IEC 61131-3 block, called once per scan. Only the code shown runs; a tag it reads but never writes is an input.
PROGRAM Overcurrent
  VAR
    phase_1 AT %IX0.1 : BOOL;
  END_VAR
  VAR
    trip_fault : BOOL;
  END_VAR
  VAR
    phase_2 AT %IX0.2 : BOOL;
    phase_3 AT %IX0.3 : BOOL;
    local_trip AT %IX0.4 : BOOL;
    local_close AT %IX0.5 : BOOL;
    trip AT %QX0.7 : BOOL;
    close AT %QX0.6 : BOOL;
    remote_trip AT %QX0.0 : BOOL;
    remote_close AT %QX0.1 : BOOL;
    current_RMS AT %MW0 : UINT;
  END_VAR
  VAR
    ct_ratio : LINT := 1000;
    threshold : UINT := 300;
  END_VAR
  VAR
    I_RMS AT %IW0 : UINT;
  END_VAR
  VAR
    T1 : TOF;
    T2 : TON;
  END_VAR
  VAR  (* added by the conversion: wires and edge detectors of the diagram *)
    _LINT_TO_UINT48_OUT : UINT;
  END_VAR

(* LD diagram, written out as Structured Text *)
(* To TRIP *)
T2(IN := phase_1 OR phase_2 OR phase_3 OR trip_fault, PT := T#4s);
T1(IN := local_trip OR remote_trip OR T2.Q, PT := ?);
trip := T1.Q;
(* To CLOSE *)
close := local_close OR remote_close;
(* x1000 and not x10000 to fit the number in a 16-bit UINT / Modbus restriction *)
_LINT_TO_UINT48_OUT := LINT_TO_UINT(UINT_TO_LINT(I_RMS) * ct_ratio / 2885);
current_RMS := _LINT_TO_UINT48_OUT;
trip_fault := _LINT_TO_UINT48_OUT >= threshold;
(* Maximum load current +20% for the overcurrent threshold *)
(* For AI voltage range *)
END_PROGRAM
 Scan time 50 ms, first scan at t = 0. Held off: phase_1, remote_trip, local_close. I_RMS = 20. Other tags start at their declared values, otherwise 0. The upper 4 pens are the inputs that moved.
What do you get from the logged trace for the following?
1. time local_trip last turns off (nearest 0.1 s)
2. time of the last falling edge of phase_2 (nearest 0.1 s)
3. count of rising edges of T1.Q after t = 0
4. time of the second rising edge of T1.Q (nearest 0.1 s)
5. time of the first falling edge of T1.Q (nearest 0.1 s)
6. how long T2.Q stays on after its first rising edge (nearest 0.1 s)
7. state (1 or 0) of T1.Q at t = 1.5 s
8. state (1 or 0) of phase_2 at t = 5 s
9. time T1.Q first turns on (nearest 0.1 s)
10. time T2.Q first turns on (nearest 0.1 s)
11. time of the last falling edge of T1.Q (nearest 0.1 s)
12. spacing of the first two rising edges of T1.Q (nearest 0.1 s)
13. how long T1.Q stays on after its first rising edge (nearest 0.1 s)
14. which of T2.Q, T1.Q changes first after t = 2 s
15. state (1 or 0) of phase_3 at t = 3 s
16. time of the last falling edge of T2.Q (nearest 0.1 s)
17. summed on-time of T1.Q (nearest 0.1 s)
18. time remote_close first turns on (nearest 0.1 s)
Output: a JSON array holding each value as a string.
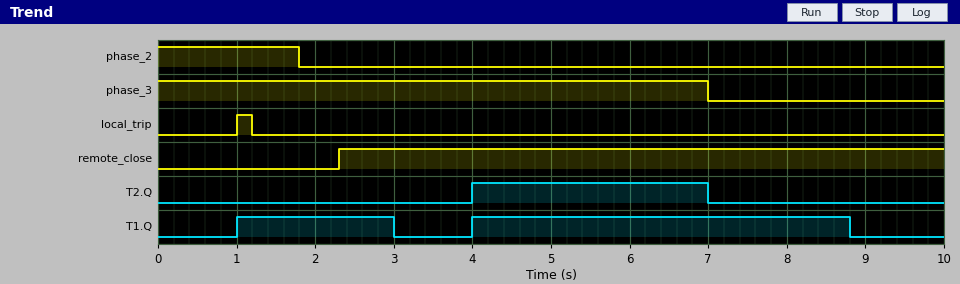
["1.2 s", "1.8 s", "2", "4.0 s", "3.0 s", "3.0 s", "1", "0", "1.0 s", "4.0 s", "8.8 s", "3.0 s", "2.0 s", "T1.Q", "1", "7.0 s", "6.8 s", "2.3 s"]
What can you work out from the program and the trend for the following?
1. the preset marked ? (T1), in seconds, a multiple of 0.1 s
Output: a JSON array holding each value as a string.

["1.8 s"]
